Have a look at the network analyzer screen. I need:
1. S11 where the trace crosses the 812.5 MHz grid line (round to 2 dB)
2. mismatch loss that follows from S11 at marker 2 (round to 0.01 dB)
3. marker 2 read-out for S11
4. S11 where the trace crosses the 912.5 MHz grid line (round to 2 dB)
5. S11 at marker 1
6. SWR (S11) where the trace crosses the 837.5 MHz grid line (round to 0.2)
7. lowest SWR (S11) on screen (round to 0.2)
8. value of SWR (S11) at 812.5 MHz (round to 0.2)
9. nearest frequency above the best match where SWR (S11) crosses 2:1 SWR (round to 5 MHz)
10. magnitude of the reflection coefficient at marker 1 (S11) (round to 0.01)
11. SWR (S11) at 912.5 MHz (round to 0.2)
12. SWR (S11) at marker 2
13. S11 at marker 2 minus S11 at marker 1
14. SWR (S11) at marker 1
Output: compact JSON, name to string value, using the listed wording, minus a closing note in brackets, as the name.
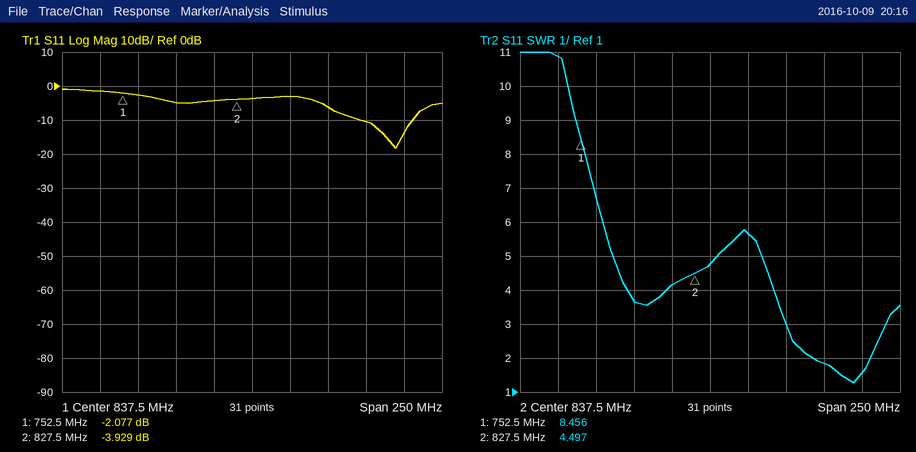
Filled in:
{"S11 where the trace crosses the 812.5 MHz grid line": "-4 dB", "mismatch loss that follows from S11 at marker 2": "2.25 dB", "marker 2 read-out for S11": "-3.929 dB", "S11 where the trace crosses the 912.5 MHz grid line": "-10 dB", "S11 at marker 1": "-2.077 dB", "SWR (S11) where the trace crosses the 837.5 MHz grid line": "4.8", "lowest SWR (S11) on screen": "1.2", "value of SWR (S11) at 812.5 MHz": "4.2", "nearest frequency above the best match where SWR (S11) crosses 2:1 SWR": "945 MHz", "magnitude of the reflection coefficient at marker 1 (S11)": "0.79", "SWR (S11) at 912.5 MHz": "1.8", "SWR (S11) at marker 2": "4.497", "S11 at marker 2 minus S11 at marker 1": "-1.852 dB", "SWR (S11) at marker 1": "8.456"}
